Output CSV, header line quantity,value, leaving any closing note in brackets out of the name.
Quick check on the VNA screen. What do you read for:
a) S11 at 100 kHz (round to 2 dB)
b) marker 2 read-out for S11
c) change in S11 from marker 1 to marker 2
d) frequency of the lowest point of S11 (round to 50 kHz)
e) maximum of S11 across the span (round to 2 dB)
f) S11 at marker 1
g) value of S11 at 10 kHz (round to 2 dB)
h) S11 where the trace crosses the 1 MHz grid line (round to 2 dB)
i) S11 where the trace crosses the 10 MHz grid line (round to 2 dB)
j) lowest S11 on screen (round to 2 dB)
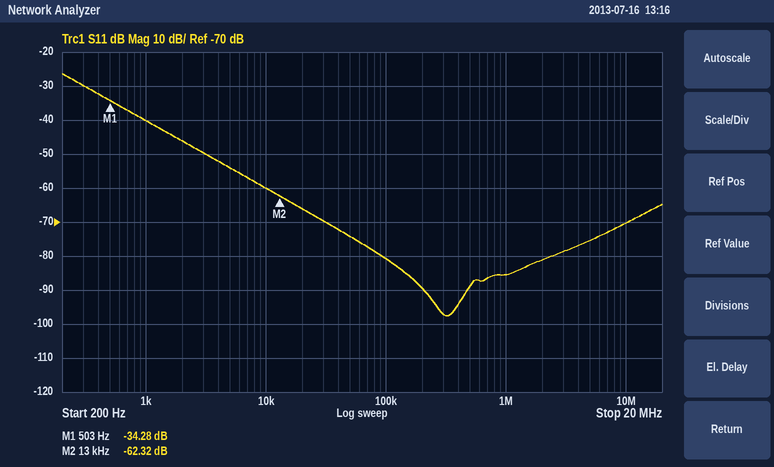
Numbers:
quantity,value
S11 at 100 kHz,-80 dB
marker 2 read-out for S11,-62.32 dB
change in S11 from marker 1 to marker 2,-28.04 dB
frequency of the lowest point of S11,300 kHz
maximum of S11 across the span,-26 dB
S11 at marker 1,-34.28 dB
value of S11 at 10 kHz,-60 dB
S11 where the trace crosses the 1 MHz grid line,-86 dB
S11 where the trace crosses the 10 MHz grid line,-70 dB
lowest S11 on screen,-98 dB
